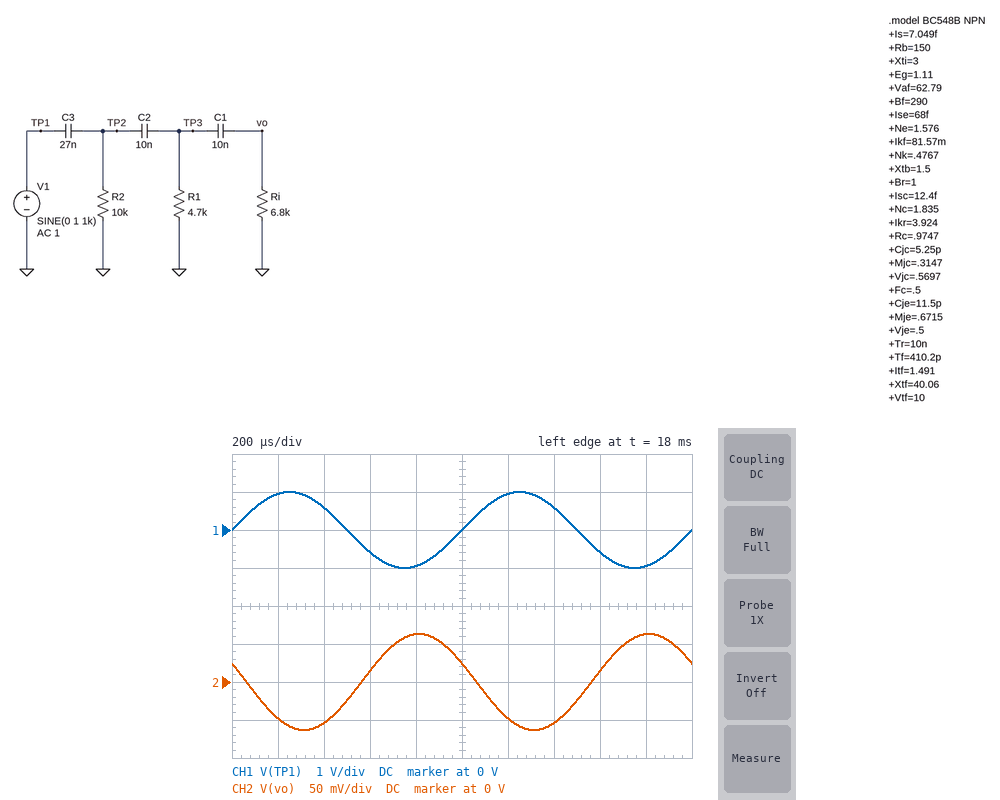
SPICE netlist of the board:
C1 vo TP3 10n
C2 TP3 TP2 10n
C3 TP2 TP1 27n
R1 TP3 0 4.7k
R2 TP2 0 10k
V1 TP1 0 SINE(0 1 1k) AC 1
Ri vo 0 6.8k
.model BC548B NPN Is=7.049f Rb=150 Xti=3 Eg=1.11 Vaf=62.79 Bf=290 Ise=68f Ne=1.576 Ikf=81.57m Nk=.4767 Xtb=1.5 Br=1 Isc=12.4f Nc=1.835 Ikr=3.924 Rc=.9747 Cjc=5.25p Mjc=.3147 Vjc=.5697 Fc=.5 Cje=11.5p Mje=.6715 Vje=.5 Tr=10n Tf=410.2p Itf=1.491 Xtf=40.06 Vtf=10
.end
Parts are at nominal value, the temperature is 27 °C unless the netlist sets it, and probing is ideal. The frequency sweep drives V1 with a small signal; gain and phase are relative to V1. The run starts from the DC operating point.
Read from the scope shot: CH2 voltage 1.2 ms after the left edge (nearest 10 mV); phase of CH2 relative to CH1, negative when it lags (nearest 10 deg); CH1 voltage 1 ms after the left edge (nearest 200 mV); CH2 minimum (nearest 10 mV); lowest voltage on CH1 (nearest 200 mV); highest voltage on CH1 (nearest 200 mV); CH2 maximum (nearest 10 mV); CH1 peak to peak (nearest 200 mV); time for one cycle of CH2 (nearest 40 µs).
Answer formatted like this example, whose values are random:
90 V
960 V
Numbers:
-50 mV
160 deg
0 V
-60 mV
-1.0 V
1.0 V
60 mV
2.0 V
1.00 ms
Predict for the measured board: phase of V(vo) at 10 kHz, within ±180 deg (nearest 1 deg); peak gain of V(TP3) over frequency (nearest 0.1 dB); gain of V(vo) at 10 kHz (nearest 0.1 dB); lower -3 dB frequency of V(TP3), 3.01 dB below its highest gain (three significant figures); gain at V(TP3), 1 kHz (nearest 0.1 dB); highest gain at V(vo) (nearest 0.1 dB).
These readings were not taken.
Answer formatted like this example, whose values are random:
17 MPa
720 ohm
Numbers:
52 deg
0 dB
-2.7 dB
8.71 kHz
-15.9 dB
0 dB
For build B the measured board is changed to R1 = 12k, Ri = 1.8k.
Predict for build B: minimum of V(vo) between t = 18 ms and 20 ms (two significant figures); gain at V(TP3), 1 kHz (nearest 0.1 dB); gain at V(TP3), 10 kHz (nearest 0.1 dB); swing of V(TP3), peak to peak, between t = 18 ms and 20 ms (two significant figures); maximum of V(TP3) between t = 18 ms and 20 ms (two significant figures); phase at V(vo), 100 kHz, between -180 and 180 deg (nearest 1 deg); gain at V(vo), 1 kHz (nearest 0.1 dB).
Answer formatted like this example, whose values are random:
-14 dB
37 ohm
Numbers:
-32 mV
-10.8 dB
-5.2 dB
570 mV
290 mV
13 deg
-29.8 dB
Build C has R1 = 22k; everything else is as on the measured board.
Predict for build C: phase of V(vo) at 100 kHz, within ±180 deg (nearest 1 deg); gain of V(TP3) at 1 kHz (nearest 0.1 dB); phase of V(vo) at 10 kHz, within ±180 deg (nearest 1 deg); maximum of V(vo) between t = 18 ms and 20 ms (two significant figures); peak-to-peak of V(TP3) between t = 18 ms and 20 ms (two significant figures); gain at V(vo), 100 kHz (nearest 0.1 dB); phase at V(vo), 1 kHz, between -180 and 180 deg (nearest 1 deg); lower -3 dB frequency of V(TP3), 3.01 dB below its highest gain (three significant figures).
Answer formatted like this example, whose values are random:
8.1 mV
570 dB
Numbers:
4 deg
-9.5 dB
37 deg
130 mV
670 mV
0 dB
126 deg
5.42 kHz
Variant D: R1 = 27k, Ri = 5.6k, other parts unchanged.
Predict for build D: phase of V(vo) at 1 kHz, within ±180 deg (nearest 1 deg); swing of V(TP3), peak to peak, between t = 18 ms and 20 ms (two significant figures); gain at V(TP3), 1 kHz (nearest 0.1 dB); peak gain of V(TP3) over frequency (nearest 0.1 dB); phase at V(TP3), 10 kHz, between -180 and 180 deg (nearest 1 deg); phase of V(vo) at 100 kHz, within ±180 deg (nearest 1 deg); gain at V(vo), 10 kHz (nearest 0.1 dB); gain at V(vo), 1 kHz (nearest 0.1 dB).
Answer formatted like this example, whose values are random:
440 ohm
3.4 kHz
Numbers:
125 deg
690 mV
-9.2 dB
0 dB
25 deg
5 deg
-1.9 dB
-18.8 dB
